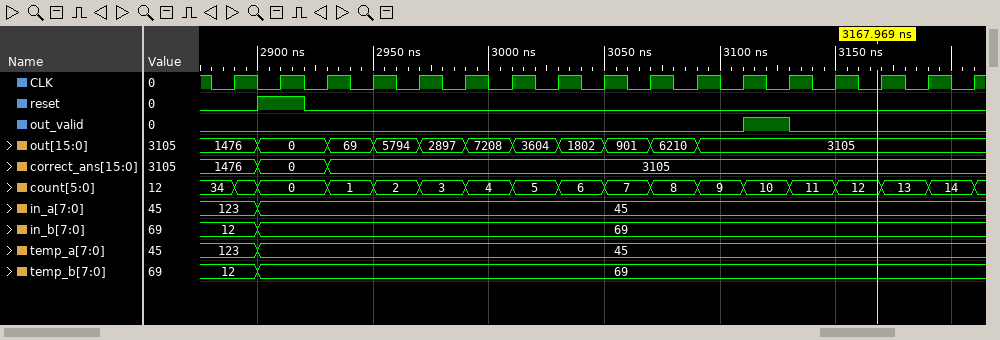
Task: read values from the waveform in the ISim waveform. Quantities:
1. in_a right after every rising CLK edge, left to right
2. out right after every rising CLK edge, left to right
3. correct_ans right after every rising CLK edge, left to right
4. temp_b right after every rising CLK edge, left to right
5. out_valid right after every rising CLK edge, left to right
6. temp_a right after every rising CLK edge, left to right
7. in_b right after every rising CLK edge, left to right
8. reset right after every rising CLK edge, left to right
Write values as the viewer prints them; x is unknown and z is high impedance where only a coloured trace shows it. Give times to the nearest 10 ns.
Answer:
123, 45, 45, 45, 45, 45, 45, 45, 45, 45, 45, 45, 45, 45, 45, 45, 45
1476, 0, 69, 5794, 2897, 7208, 3604, 1802, 901, 6210, 3105, 3105, 3105, 3105, 3105, 3105, 3105
1476, 0, 3105, 3105, 3105, 3105, 3105, 3105, 3105, 3105, 3105, 3105, 3105, 3105, 3105, 3105, 3105
12, 69, 69, 69, 69, 69, 69, 69, 69, 69, 69, 69, 69, 69, 69, 69, 69
0 0 0 0 0 0 0 0 0 0 0 1 0 0 0 0 0
123, 45, 45, 45, 45, 45, 45, 45, 45, 45, 45, 45, 45, 45, 45, 45, 45
12, 69, 69, 69, 69, 69, 69, 69, 69, 69, 69, 69, 69, 69, 69, 69, 69
0 1 0 0 0 0 0 0 0 0 0 0 0 0 0 0 0
